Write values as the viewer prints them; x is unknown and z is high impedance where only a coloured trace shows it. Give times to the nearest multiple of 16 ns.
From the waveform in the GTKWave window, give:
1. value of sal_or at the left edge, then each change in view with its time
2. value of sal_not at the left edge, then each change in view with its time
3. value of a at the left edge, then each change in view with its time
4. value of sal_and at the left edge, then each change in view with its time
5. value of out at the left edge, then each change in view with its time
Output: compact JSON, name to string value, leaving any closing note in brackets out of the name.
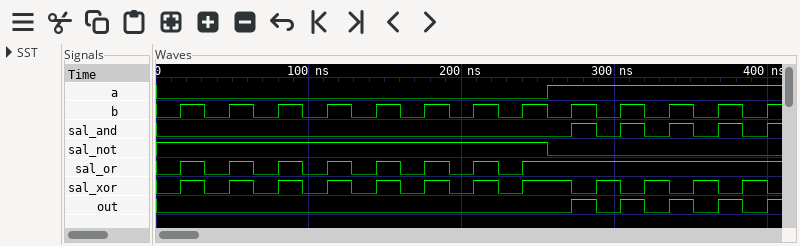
{"value of sal_or at the left edge, then each change in view with its time": "0, 1 at 16 ns, 0 at 32 ns, 1 at 48 ns, 0 at 64 ns, 1 at 80 ns, 0 at 96 ns, 1 at 112 ns, 0 at 128 ns, 1 at 144 ns, 0 at 160 ns, 1 at 176 ns, 0 at 192 ns, 1 at 208 ns, 0 at 224 ns, 1 at 240 ns", "value of sal_not at the left edge, then each change in view with its time": "1, 0 at 256 ns", "value of a at the left edge, then each change in view with its time": "0, 1 at 256 ns", "value of sal_and at the left edge, then each change in view with its time": "0, 1 at 272 ns, 0 at 288 ns, 1 at 304 ns, 0 at 320 ns, 1 at 336 ns, 0 at 352 ns, 1 at 368 ns, 0 at 384 ns, 1 at 400 ns", "value of out at the left edge, then each change in view with its time": "0, 1 at 272 ns, 0 at 288 ns, 1 at 304 ns, 0 at 320 ns, 1 at 336 ns, 0 at 352 ns, 1 at 368 ns, 0 at 384 ns, 1 at 400 ns"}
